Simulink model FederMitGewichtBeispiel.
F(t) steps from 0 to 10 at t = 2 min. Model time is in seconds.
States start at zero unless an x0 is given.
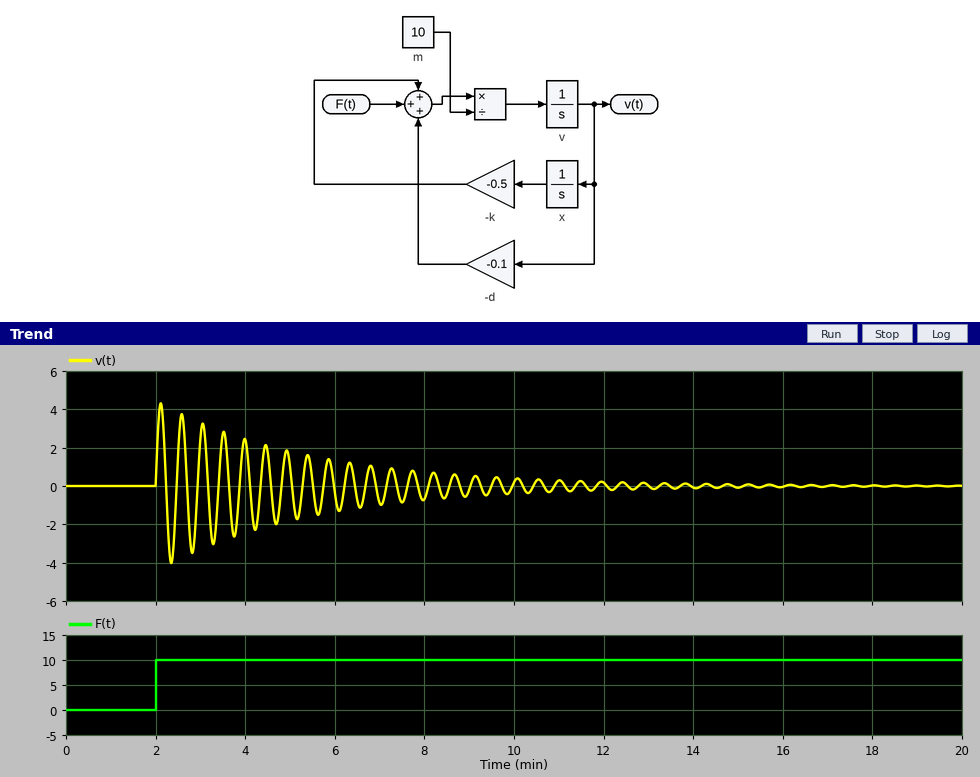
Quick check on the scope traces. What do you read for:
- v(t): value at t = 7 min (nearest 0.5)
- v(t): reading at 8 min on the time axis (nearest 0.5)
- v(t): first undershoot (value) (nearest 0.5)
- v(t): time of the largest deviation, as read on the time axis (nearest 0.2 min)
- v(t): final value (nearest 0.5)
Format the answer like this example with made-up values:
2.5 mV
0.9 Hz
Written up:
-1.0
-0.5
-4.0
2.2 min
0.0
